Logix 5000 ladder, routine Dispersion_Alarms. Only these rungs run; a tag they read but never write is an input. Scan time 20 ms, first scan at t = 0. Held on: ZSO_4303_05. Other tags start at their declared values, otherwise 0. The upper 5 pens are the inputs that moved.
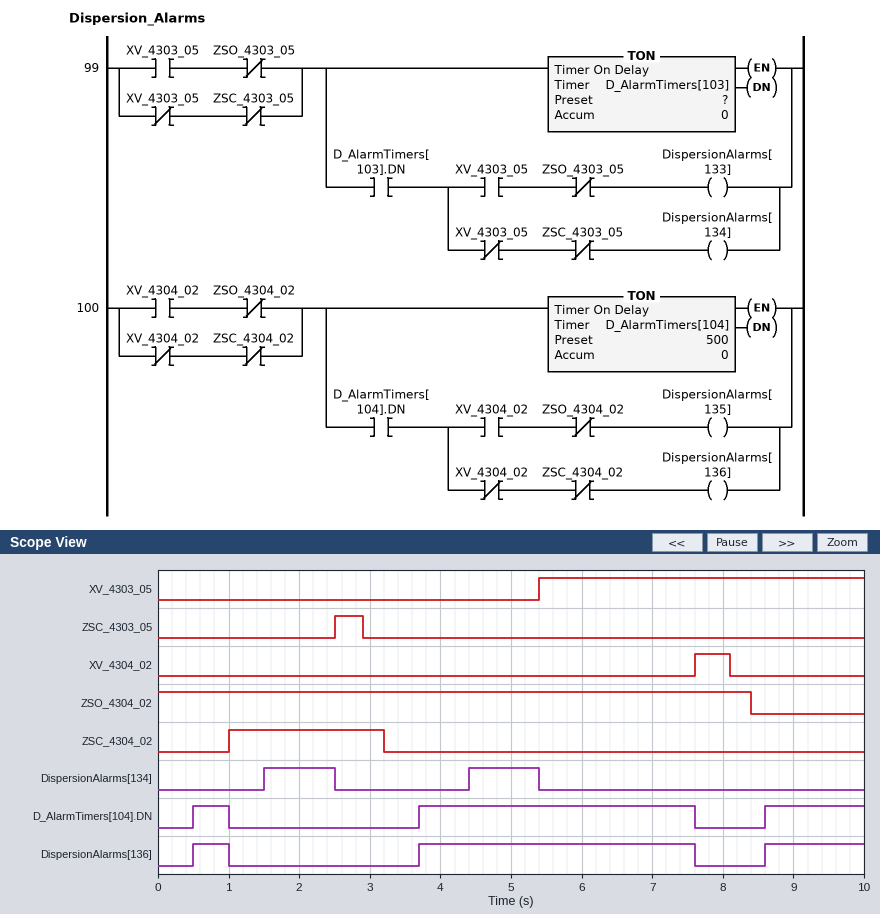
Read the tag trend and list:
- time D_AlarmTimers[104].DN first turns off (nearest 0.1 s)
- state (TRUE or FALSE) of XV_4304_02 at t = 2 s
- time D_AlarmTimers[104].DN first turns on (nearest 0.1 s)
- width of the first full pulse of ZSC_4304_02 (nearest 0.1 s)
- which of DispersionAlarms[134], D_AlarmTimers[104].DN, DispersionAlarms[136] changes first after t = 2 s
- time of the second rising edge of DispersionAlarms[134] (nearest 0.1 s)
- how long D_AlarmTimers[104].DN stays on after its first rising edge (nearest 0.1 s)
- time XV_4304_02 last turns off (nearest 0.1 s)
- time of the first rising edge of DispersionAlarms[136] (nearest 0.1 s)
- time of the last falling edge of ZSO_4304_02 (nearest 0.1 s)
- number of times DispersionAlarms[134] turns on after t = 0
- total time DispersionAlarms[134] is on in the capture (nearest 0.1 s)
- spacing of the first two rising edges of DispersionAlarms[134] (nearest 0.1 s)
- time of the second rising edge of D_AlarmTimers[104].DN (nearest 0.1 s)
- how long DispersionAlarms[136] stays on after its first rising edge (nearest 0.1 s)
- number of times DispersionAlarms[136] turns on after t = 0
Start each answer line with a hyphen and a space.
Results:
- 1.0 s
- FALSE
- 0.5 s
- 2.2 s
- DispersionAlarms[134]
- 4.4 s
- 0.5 s
- 8.1 s
- 0.5 s
- 8.4 s
- 2
- 2.0 s
- 2.9 s
- 3.7 s
- 0.5 s
- 3
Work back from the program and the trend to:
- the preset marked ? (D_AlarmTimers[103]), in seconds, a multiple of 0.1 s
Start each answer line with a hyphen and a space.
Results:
- 1.5 s
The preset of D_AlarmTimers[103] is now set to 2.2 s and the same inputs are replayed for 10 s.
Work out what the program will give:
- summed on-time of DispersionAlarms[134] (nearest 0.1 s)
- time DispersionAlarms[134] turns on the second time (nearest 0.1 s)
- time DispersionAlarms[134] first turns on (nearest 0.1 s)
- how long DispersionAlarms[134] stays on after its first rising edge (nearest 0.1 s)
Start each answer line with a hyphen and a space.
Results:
- 0.6 s
- 5.1 s
- 2.2 s
- 0.3 s
